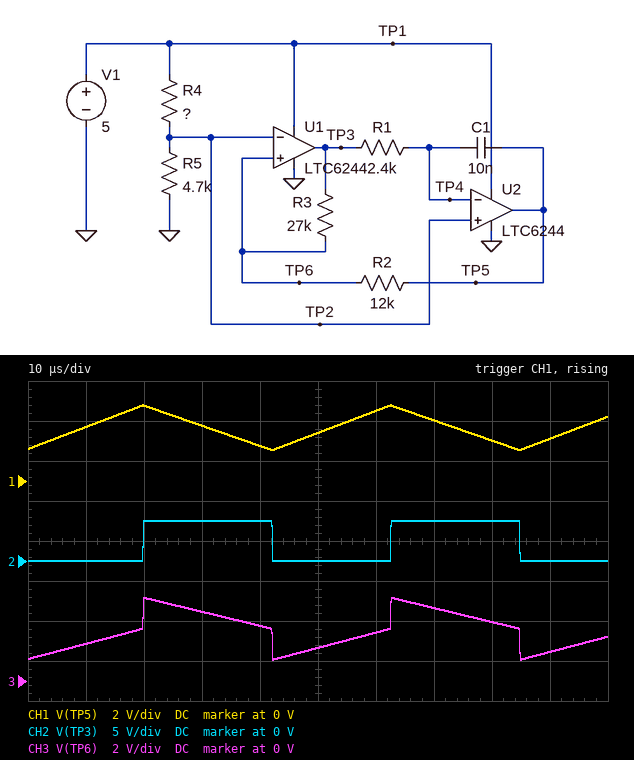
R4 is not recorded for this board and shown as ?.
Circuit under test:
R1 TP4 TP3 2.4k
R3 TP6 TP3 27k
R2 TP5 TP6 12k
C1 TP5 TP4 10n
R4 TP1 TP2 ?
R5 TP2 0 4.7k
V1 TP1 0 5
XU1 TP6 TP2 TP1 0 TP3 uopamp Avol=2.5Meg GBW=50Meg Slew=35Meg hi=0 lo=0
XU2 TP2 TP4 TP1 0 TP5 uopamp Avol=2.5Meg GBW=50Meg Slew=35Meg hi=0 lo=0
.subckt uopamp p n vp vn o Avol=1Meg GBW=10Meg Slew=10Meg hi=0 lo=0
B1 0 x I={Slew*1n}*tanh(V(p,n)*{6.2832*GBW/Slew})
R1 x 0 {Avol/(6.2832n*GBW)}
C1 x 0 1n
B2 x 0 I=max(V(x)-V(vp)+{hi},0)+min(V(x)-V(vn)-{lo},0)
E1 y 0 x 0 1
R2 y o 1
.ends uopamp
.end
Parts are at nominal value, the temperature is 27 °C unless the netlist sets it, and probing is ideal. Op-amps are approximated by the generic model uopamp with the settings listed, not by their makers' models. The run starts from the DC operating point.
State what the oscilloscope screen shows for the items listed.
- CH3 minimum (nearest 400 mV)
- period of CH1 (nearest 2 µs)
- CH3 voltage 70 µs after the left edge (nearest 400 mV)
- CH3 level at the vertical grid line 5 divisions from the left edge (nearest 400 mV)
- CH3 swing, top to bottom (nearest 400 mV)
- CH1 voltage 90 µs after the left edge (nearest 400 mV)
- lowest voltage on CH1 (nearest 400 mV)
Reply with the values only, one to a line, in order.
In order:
1.2 V
42 µs
3.6 V
1.6 V
3.2 V
2.0 V
1.6 V
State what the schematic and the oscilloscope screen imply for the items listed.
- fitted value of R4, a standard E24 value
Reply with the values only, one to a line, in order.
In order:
4.3 kΩ
